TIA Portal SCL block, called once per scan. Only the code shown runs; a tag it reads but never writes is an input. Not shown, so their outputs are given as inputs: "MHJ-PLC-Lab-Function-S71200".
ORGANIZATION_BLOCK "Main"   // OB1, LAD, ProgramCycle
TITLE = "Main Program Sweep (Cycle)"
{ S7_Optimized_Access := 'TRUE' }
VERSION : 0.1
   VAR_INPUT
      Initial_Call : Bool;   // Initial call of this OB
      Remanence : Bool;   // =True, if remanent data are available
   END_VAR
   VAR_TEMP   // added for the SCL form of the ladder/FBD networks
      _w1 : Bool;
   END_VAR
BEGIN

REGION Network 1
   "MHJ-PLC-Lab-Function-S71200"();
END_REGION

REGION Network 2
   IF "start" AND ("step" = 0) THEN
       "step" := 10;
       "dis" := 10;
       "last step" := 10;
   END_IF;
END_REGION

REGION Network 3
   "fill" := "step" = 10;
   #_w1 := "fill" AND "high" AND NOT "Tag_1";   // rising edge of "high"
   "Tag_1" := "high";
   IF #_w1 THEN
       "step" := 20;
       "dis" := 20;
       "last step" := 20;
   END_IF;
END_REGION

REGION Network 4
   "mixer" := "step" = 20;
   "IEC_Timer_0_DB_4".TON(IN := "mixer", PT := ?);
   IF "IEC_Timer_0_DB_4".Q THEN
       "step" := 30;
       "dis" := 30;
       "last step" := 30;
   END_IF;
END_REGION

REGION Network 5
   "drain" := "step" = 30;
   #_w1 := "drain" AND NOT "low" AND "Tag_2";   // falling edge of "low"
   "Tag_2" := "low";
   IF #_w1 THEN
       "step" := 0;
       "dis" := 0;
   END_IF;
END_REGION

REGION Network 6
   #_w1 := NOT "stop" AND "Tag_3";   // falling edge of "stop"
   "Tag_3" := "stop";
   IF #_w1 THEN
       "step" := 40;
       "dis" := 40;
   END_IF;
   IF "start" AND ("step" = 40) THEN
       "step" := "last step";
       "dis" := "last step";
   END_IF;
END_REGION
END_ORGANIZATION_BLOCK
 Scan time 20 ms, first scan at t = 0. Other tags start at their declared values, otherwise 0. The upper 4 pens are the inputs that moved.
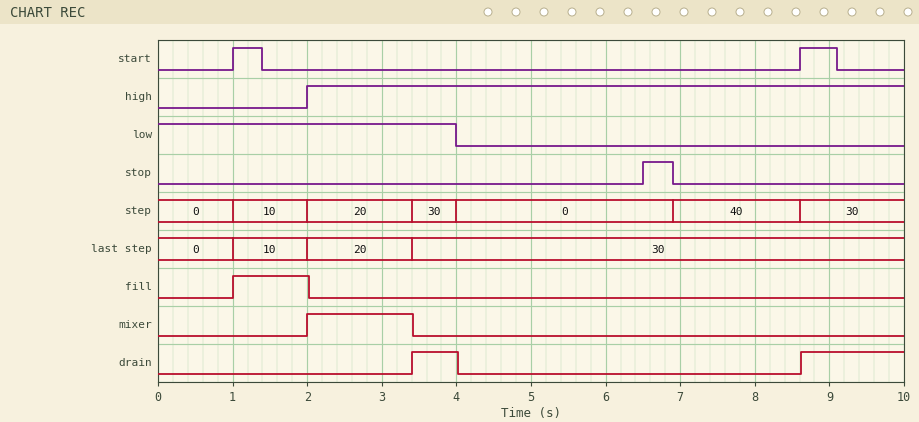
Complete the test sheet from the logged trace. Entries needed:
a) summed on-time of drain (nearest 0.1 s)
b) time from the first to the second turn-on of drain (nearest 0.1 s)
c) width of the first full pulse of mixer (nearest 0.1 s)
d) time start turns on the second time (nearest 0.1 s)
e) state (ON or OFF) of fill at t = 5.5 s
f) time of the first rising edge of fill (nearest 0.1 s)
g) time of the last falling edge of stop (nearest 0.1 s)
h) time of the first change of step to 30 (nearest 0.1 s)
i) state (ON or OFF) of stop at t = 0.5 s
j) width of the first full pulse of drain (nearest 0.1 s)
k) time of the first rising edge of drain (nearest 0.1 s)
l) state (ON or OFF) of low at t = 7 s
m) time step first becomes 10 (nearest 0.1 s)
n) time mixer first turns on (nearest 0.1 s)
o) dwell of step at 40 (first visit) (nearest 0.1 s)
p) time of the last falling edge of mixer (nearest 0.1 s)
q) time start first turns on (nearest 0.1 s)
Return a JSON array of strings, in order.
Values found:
["2.0 s", "5.2 s", "1.4 s", "8.6 s", "OFF", "1.0 s", "6.9 s", "3.4 s", "OFF", "0.6 s", "3.4 s", "OFF", "1.0 s", "2.0 s", "1.7 s", "3.4 s", "1.0 s"]
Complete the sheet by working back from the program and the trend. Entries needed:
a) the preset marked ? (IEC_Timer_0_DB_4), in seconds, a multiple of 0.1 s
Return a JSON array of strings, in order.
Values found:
["1.4 s"]
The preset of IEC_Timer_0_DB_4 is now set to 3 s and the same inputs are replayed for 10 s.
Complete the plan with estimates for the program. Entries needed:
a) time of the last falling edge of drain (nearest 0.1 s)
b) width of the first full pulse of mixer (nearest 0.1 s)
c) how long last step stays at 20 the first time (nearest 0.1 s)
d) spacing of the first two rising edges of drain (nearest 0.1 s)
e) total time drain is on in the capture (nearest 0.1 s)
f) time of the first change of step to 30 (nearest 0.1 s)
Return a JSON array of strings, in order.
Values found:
["6.9 s", "3.0 s", "3.0 s", "3.6 s", "3.3 s", "5.0 s"]
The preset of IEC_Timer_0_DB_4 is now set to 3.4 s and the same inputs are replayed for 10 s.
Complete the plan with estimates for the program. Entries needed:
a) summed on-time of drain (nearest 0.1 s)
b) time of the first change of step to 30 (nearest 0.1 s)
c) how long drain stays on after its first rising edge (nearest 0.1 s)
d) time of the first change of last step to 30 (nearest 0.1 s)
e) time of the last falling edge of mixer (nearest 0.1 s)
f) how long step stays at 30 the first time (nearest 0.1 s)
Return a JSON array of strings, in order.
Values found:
["2.9 s", "5.4 s", "1.5 s", "5.4 s", "5.4 s", "1.5 s"]
